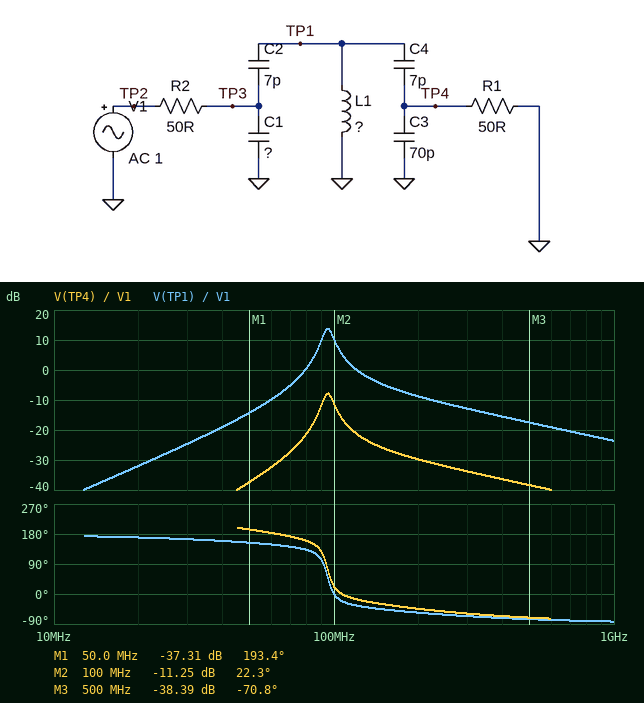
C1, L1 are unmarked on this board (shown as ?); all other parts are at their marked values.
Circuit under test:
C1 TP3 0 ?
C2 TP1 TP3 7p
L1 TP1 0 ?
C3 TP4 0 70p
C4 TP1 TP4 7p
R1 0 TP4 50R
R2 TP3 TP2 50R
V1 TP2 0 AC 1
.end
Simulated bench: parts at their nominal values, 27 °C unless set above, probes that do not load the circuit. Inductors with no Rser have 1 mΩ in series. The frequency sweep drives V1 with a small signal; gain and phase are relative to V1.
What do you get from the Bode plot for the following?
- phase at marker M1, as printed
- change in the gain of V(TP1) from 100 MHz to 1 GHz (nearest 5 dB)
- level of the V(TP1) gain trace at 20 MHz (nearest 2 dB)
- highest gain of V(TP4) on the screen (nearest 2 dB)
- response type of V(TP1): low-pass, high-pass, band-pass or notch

193.4 deg
-35 dB
-32 dB
-8 dB
band-pass
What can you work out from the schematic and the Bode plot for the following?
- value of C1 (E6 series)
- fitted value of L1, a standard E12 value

22 pF
220 nH
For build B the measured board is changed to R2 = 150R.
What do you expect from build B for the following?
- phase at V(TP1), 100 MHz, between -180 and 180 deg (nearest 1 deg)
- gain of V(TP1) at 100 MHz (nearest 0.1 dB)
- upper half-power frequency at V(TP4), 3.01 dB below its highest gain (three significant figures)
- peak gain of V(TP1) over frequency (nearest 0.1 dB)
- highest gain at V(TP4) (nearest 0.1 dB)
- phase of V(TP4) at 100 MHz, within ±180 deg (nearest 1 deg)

-10 deg
8.6 dB
101 MHz
9.9 dB
-11.6 dB
12 deg
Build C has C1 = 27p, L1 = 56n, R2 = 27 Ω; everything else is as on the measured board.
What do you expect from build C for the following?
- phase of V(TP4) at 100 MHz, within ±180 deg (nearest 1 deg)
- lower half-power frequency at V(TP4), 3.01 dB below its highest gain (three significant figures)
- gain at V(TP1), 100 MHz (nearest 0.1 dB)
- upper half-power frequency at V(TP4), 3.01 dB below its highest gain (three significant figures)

171 deg
183 MHz
-14.5 dB
196 MHz
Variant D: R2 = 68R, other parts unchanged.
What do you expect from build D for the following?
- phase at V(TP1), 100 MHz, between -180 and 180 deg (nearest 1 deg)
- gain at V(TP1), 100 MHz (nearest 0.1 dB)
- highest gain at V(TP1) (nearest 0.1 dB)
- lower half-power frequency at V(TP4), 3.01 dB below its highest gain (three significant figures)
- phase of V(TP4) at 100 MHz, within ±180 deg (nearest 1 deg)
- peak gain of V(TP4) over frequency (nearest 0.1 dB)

-2 deg
10.0 dB
12.5 dB
92.0 MHz
20 deg
-9.0 dB
